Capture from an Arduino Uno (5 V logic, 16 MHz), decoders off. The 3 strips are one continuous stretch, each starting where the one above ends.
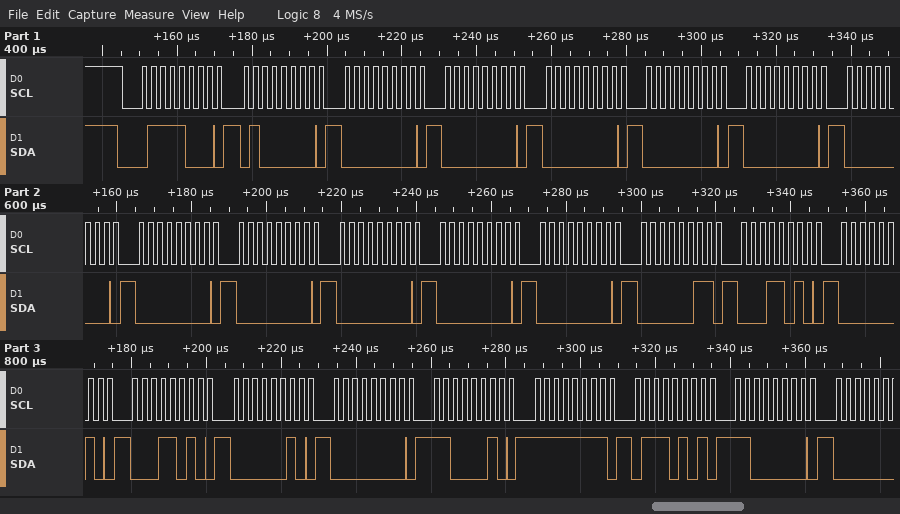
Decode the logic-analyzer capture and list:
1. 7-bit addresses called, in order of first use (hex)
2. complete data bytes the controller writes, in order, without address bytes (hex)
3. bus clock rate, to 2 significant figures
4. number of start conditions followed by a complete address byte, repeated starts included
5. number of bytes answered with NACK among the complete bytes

0x3C
40 00 00 00 00 00 00 00 00 00 00 00 03 1A 02 1A 02 00 C2 FF 75 C0
400 kHz
1
0
